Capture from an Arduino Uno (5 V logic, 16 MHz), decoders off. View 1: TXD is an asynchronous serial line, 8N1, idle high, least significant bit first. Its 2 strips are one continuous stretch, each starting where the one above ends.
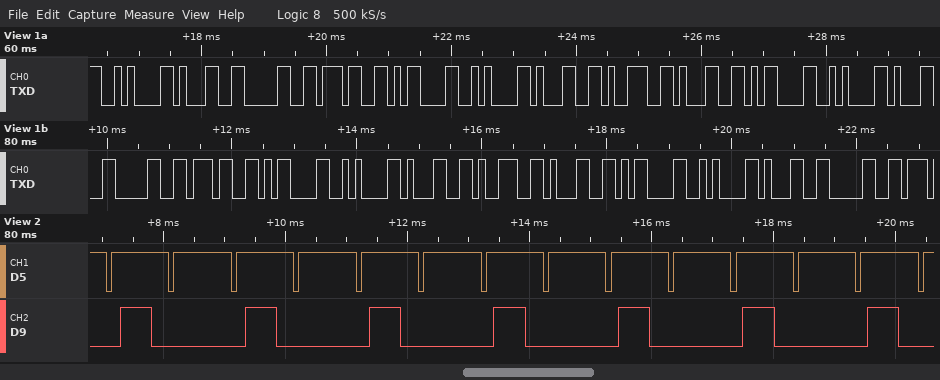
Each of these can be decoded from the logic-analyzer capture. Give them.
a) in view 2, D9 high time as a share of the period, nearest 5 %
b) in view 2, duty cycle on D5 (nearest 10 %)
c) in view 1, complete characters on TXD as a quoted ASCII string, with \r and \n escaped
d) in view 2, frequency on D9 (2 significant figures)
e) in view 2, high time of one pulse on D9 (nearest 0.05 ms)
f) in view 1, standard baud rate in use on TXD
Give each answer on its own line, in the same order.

25 %
90 %
"\n107\r\n191\r\n107\r\n191\r\n10"
490 Hz
0.50 ms
9600 baud
